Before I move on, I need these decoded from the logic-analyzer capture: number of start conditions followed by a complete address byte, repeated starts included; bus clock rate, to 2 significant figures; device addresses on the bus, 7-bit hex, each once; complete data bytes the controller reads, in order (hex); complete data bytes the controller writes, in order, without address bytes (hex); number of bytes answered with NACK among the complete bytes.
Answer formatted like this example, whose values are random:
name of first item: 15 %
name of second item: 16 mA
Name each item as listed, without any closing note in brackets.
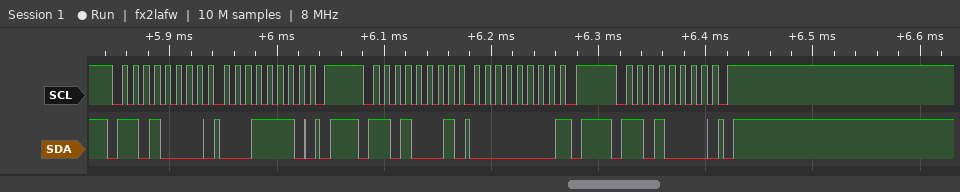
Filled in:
number of start conditions followed by a complete address byte, repeated starts included: 3
bus clock rate, to 2 significant figures: 100 kHz
device addresses on the bus, 7-bit hex, each once: 0x68
complete data bytes the controller reads, in order: 00
complete data bytes the controller writes, in order, without address bytes: 1E
number of bytes answered with NACK among the complete bytes: 1
